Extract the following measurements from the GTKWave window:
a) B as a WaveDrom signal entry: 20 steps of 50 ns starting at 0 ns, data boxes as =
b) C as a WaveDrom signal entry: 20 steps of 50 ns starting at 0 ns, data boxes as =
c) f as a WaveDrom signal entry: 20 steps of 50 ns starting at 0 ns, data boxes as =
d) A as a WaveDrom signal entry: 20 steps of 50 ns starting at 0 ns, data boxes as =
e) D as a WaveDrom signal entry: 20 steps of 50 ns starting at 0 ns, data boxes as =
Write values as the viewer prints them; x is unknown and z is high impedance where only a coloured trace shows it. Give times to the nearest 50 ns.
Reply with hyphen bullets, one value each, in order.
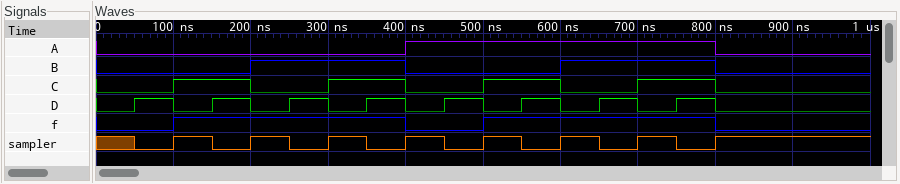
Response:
- {name: 'B', wave: '0...1...0...1...0...'}
- {name: 'C', wave: '0.1.0.1.0.1.0.1.0...'}
- {name: 'f', wave: '0.1.....0.1.....0...'}
- {name: 'A', wave: '0.......1.......0...'}
- {name: 'D', wave: '01010101010101010...'}
